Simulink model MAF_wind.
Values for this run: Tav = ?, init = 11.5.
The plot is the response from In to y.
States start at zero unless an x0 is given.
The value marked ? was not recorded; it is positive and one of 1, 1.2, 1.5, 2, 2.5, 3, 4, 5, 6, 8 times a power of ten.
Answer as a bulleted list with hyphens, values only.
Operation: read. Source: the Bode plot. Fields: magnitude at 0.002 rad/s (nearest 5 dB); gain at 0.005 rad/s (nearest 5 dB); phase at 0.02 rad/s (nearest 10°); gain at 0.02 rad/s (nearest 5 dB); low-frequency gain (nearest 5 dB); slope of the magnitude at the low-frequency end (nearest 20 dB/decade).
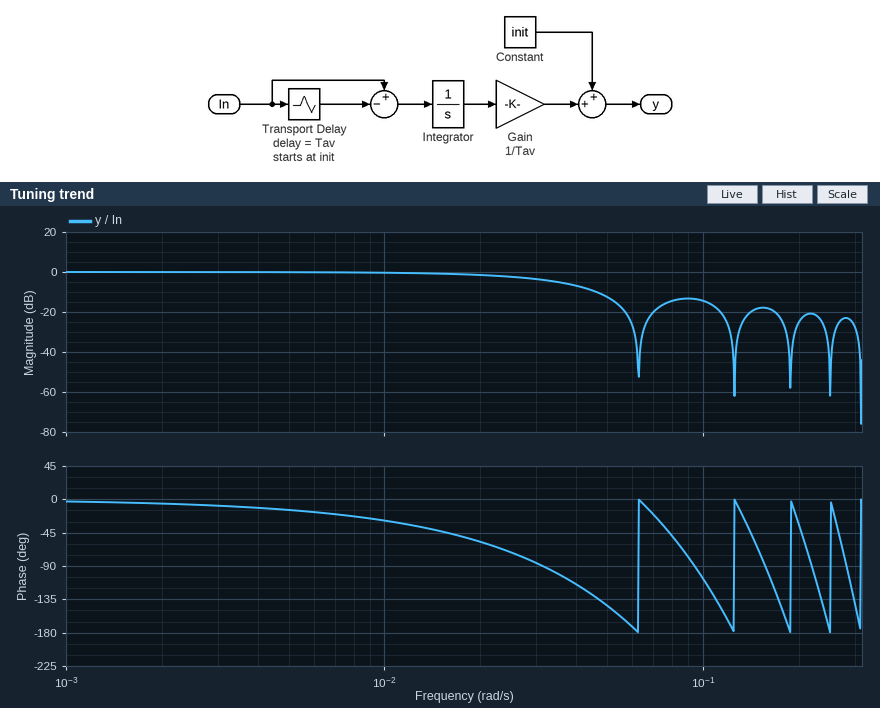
- 0 dB
- 0 dB
- -60°
- 0 dB
- 0 dB
- 0 dB/decade
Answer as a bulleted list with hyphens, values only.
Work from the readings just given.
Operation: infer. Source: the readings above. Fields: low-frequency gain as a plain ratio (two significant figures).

- 1.0
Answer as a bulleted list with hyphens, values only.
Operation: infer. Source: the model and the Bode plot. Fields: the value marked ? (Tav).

- 100
